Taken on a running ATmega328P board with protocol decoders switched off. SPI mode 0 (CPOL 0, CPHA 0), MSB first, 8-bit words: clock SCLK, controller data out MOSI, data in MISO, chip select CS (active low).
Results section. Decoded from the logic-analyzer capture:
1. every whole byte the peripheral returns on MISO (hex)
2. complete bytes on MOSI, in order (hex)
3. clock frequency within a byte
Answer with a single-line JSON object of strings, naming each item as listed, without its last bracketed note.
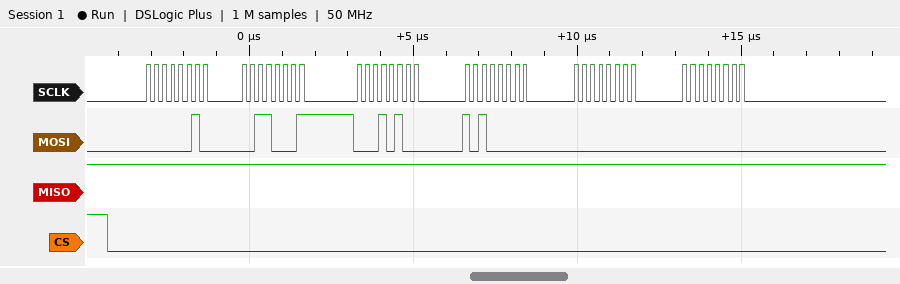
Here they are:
{"every whole byte the peripheral returns on MISO": "FF FF FF FF FF FF", "complete bytes on MOSI, in order": "02 31 14 A0 00 00", "clock frequency within a byte": "4 MHz"}
